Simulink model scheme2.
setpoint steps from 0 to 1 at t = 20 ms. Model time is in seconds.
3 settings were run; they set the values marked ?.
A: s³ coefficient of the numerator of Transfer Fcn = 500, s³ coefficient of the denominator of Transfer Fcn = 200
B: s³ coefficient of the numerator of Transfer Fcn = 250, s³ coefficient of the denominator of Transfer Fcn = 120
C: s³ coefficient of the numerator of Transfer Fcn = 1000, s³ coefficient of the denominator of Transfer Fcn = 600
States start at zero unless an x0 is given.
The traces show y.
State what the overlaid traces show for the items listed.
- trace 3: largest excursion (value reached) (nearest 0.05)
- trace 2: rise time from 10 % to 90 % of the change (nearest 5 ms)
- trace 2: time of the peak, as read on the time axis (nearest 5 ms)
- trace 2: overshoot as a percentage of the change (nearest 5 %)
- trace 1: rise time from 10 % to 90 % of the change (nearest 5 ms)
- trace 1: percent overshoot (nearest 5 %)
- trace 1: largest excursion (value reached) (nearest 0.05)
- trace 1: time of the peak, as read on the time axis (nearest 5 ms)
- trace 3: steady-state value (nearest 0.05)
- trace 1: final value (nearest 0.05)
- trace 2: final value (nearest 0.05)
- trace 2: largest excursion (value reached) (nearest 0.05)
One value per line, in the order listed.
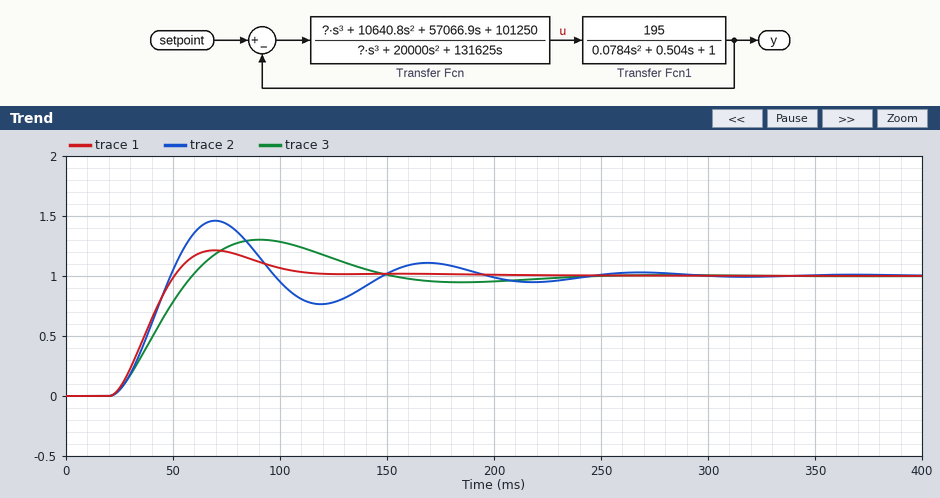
1.30
20 ms
70 ms
45 %
20 ms
20 %
1.20
70 ms
1.00
1.00
1.00
1.45
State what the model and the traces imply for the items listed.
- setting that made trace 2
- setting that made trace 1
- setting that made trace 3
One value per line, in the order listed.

C
A
B
